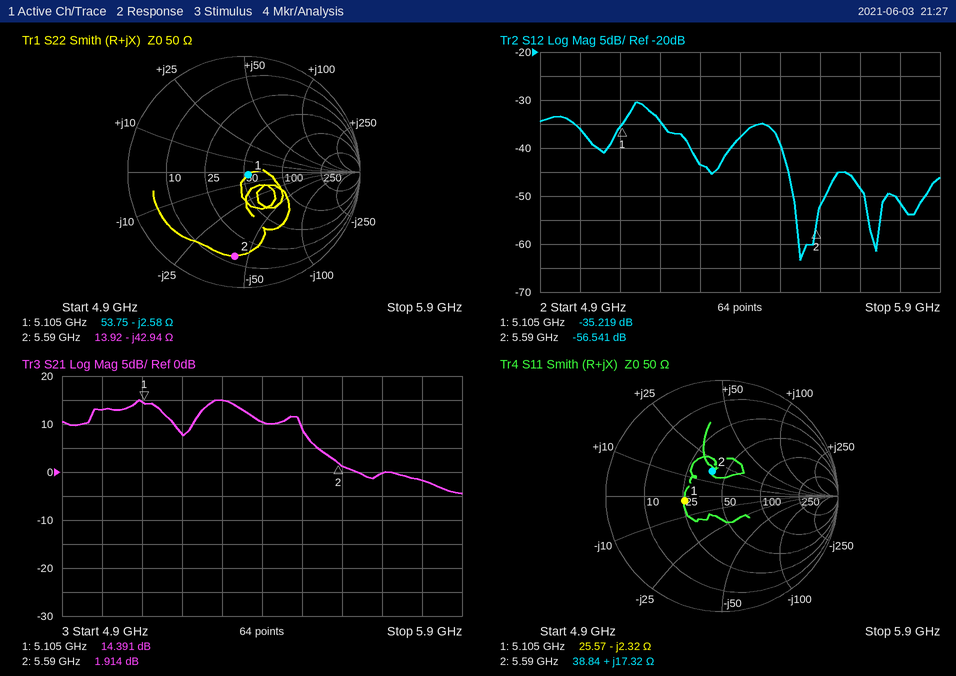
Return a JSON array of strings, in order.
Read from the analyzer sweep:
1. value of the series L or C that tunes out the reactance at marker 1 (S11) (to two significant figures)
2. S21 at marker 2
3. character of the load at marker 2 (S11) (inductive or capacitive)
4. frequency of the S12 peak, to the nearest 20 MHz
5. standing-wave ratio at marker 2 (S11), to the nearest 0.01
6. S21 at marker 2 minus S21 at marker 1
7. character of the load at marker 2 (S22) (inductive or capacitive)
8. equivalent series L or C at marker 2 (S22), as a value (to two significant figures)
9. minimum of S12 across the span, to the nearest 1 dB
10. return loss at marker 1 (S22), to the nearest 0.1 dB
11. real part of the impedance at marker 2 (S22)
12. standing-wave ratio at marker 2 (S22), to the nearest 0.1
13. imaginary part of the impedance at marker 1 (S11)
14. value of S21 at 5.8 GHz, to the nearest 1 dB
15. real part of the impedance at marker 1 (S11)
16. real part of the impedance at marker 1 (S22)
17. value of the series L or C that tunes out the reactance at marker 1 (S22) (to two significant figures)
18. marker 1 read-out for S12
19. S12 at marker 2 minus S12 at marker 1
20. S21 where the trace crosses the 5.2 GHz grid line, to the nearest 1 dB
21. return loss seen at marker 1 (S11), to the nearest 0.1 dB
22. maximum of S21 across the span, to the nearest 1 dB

["72 pH", "1.914 dB", "inductive", "5.14 GHz", "1.59", "-12.477 dB", "capacitive", "660 fF", "-63 dB", "27.2 dB", "13.92 Ω", "6.4", "-2.32 Ω", "-2 dB", "25.57 Ω", "53.75 Ω", "80 pH", "-35.219 dB", "-21.322 dB", "8 dB", "9.8 dB", "15 dB"]
